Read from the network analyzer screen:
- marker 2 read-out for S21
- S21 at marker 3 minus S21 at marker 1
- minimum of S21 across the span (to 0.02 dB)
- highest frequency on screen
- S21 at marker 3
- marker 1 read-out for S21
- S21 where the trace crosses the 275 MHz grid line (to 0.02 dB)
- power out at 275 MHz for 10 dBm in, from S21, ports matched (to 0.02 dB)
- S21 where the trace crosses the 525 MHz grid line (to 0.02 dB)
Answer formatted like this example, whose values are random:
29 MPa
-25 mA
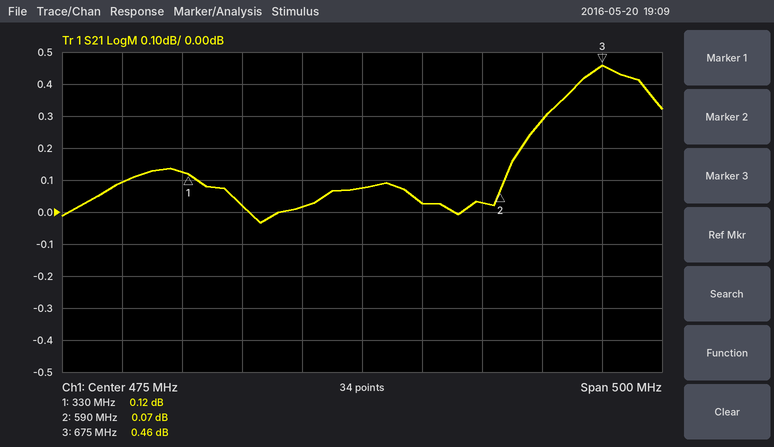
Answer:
0.07 dB
0.34 dB
-0.04 dB
725 MHz
0.46 dB
0.12 dB
0.10 dB
10.10 dBm
0.02 dB
